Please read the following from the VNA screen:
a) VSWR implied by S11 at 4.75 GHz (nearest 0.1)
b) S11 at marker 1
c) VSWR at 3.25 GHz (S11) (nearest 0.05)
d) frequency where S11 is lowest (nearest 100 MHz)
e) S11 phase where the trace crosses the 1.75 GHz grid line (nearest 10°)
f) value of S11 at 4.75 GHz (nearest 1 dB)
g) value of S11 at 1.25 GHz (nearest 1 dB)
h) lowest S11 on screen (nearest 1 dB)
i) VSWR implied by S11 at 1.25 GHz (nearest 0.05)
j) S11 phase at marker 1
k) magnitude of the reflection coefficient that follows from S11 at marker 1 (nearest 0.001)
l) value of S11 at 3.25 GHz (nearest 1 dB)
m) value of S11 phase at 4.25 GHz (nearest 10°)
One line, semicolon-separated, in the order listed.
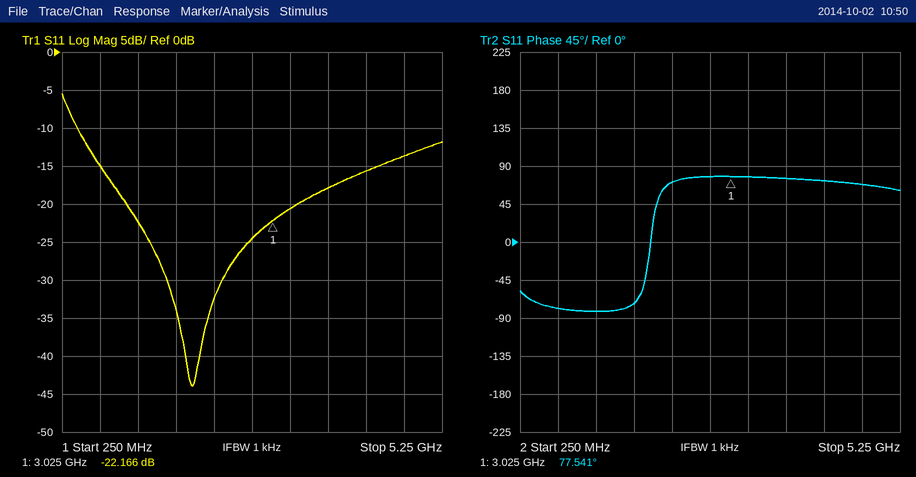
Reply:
1.5; -22.166 dB; 1.20; 2.0 GHz; -70°; -14 dB; -22 dB; -44 dB; 1.15; 77.541°; 0.078; -21 dB; 70°
